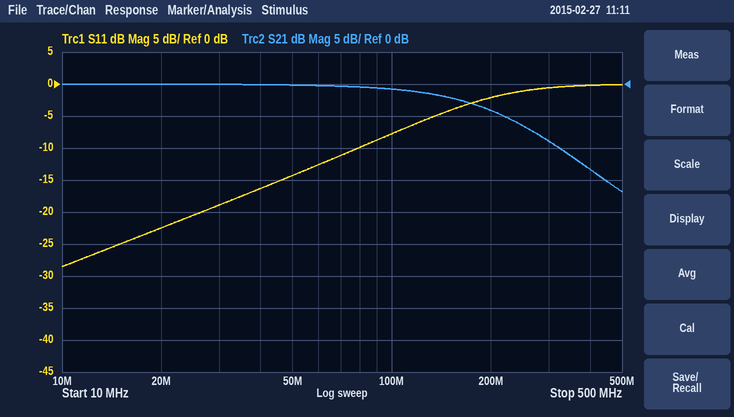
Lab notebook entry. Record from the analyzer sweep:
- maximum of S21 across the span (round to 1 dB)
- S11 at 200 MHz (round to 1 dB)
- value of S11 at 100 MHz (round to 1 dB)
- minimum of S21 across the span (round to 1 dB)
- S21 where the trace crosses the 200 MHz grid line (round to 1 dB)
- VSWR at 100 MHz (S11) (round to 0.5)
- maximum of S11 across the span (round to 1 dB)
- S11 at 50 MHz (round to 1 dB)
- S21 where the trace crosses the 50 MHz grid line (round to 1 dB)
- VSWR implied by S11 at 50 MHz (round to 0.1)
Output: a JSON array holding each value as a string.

["0 dB", "-2 dB", "-8 dB", "-17 dB", "-4 dB", "2.5", "0 dB", "-14 dB", "0 dB", "1.5"]
